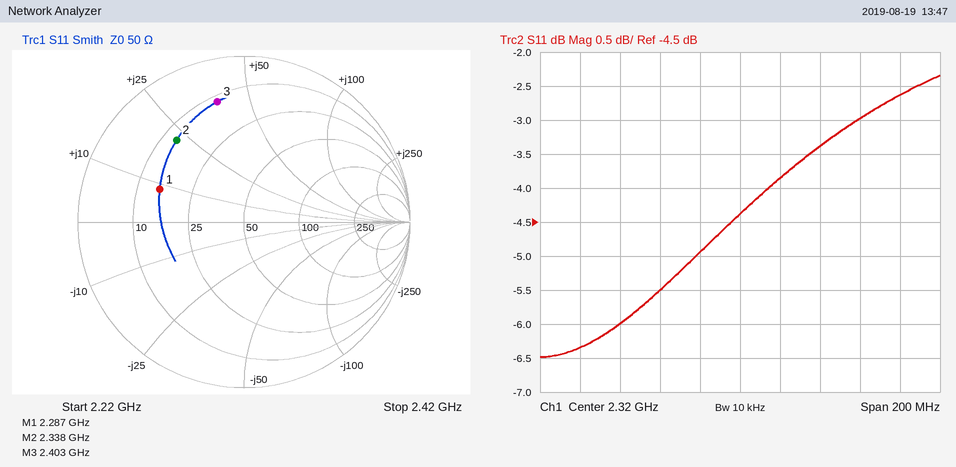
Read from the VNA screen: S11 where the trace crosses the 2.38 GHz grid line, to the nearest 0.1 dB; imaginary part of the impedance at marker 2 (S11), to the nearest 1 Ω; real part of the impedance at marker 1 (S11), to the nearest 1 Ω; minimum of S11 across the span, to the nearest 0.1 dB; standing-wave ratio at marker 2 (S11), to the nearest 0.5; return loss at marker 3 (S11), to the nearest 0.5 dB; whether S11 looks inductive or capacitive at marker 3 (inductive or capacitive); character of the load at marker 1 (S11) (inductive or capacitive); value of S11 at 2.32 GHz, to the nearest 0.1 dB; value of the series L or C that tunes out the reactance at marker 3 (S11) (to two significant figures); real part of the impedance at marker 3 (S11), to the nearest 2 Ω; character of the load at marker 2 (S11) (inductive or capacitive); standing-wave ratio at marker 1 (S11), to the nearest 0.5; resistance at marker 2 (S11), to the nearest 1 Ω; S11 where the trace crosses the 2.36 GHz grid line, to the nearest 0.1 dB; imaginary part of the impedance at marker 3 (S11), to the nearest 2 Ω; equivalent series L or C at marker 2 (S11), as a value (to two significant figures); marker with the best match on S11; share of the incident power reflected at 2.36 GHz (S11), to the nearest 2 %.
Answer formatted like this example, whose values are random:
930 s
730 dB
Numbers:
-3.0 dB
+22 Ω
15 Ω
-6.5 dB
4.5
2.5 dB
inductive
inductive
-4.4 dB
1.7 pF
12 Ω
inductive
3.5
13 Ω
-3.4 dB
+38 Ω
1.5 nH
marker 1
46 %
